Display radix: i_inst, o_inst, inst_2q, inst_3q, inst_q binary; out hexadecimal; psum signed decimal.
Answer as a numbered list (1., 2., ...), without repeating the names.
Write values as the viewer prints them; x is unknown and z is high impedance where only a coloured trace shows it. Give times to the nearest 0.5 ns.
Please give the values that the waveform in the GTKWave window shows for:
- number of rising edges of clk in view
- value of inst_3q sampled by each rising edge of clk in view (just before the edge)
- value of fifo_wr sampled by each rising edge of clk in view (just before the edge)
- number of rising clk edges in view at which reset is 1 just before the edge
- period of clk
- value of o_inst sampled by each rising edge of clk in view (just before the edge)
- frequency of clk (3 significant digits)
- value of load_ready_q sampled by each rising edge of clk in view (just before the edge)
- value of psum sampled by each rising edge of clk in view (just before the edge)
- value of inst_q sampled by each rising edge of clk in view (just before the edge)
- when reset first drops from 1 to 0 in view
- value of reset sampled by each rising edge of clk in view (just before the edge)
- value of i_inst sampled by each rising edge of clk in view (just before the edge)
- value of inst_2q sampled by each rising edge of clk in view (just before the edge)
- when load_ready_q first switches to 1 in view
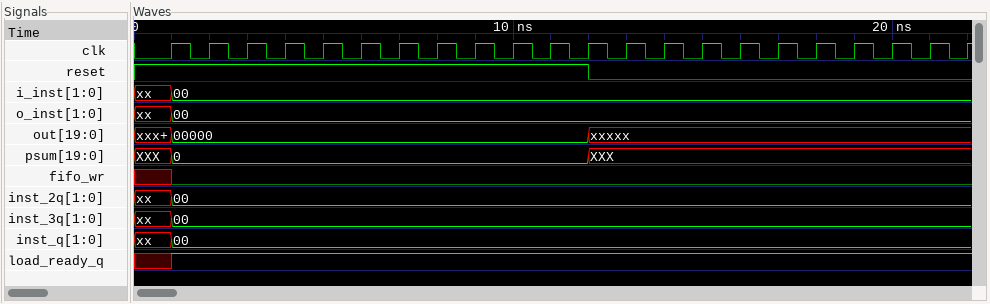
1. 22
2. xx, 00, 00, 00, 00, 00, 00, 00, 00, 00, 00, 00, 00, 00, 00, 00, 00, 00, 00, 00, 00, 00
3. x 0 0 0 0 0 0 0 0 0 0 0 0 0 0 0 0 0 0 0 0 0
4. 12
5. 1 ns
6. xx, 00, 00, 00, 00, 00, 00, 00, 00, 00, 00, 00, 00, 00, 00, 00, 00, 00, 00, 00, 00, 00
7. 1.00 GHz
8. x 1 1 1 1 1 1 1 1 1 1 1 1 1 1 1 1 1 1 1 1 1
9. XXX, 0, 0, 0, 0, 0, 0, 0, 0, 0, 0, 0, XXX, XXX, XXX, XXX, XXX, XXX, XXX, XXX, XXX, XXX
10. xx, 00, 00, 00, 00, 00, 00, 00, 00, 00, 00, 00, 00, 00, 00, 00, 00, 00, 00, 00, 00, 00
11. 12 ns
12. 1 1 1 1 1 1 1 1 1 1 1 1 0 0 0 0 0 0 0 0 0 0
13. xx, 00, 00, 00, 00, 00, 00, 00, 00, 00, 00, 00, 00, 00, 00, 00, 00, 00, 00, 00, 00, 00
14. xx, 00, 00, 00, 00, 00, 00, 00, 00, 00, 00, 00, 00, 00, 00, 00, 00, 00, 00, 00, 00, 00
15. 1 ns
